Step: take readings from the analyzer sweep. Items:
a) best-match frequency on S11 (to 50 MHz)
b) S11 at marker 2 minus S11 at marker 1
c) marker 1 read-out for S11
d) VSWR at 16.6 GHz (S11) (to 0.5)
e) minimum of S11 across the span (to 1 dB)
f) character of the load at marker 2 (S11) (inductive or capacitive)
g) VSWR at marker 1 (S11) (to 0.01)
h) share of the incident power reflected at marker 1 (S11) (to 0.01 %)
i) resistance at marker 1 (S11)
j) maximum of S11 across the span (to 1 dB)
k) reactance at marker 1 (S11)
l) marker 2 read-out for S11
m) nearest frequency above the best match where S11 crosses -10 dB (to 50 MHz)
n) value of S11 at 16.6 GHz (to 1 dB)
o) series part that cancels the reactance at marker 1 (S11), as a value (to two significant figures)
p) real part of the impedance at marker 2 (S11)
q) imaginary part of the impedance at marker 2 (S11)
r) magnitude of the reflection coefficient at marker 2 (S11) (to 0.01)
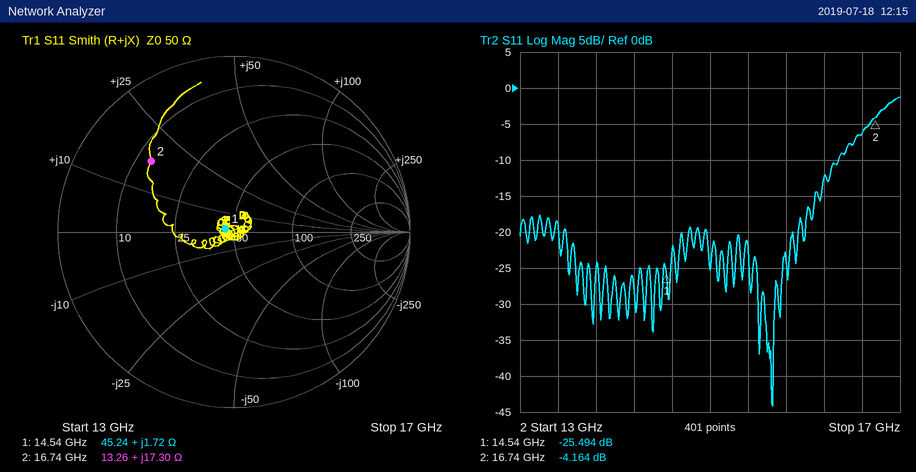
15.65 GHz
21.330 dB
-25.494 dB
3.0
-44 dB
inductive
1.11
0.28 %
45.24 Ω
-1 dB
+1.72 Ω
-4.164 dB
16.35 GHz
-6 dB
6.4 pF
13.26 Ω
+17.30 Ω
0.62
